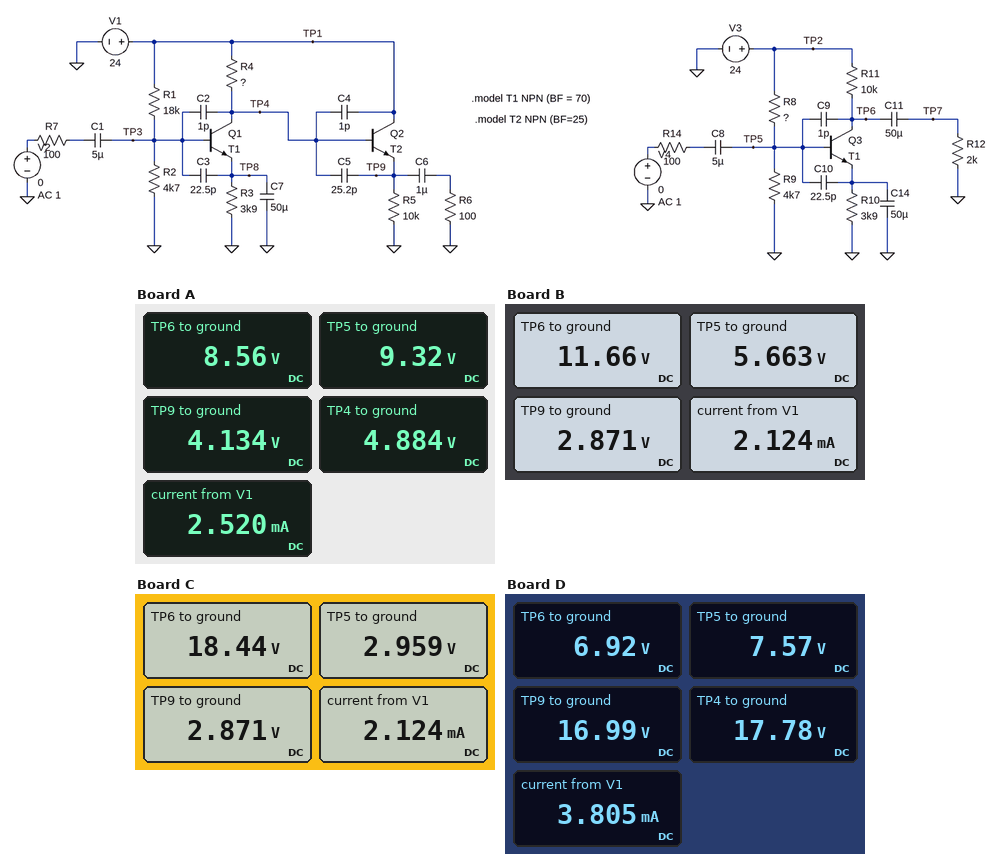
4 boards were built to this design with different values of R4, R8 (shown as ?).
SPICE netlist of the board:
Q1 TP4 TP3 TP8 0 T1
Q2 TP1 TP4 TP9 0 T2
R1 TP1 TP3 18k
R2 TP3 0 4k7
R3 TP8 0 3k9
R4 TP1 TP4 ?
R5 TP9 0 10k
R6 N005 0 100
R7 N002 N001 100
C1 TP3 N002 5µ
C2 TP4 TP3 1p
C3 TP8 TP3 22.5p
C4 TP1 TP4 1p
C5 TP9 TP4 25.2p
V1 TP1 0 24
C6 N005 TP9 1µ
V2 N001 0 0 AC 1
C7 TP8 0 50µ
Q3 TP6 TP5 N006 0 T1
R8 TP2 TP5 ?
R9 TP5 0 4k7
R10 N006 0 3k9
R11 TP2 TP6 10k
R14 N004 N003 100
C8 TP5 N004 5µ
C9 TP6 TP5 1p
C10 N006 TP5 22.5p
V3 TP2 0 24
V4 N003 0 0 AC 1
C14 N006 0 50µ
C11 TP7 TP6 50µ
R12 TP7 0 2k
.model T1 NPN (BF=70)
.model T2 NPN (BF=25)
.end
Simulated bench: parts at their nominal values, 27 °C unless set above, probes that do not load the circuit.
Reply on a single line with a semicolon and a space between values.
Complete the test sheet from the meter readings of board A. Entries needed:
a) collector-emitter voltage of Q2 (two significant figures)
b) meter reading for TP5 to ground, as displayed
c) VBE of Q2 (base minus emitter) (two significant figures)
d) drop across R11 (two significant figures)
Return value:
20 V; 9.32 V; 750 mV; 15 V
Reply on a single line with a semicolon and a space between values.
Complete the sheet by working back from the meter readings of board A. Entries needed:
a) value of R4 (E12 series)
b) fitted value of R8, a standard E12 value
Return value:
18 kΩ; 5.6 kΩ
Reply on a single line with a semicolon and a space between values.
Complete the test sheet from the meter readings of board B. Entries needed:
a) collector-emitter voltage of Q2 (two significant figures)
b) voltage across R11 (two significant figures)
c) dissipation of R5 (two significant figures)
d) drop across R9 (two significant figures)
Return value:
21 V; 12 V; 820 µW; 5.7 V
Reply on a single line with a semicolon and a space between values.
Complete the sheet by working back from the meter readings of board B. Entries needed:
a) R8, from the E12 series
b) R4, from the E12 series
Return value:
15 kΩ; 27 kΩ
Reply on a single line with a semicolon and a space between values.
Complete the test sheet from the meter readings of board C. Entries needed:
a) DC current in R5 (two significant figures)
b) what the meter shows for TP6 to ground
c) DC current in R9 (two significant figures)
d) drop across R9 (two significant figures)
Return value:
290 µA; 18.44 V; 630 µA; 3.0 V
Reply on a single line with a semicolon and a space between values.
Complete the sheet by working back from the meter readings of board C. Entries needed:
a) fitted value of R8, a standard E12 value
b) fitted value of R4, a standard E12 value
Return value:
33 kΩ; 27 kΩ
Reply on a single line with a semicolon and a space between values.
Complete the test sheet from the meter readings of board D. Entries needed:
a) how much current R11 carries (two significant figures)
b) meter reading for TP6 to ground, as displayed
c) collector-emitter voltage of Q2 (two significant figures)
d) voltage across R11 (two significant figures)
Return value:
1.7 mA; 6.92 V; 7.0 V; 17 V
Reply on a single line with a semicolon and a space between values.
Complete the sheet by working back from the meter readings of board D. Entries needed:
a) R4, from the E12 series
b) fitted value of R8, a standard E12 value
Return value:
5.6 kΩ; 10 kΩ
